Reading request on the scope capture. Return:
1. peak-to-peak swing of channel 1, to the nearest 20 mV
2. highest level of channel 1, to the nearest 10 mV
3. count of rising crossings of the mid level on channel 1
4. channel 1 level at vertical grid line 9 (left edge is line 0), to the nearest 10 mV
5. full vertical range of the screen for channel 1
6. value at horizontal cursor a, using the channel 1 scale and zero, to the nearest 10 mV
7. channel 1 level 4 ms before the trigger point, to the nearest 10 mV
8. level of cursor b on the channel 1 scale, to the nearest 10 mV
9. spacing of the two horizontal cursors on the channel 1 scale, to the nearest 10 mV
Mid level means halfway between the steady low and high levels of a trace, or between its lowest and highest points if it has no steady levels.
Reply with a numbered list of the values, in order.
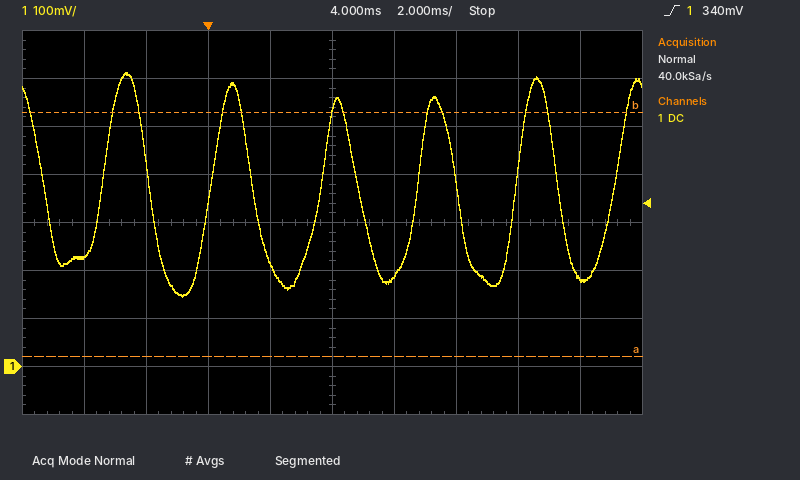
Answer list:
1. 460 mV
2. 610 mV
3. 6
4. 180 mV
5. 800 mV
6. 20 mV
7. 230 mV
8. 530 mV
9. 510 mV
